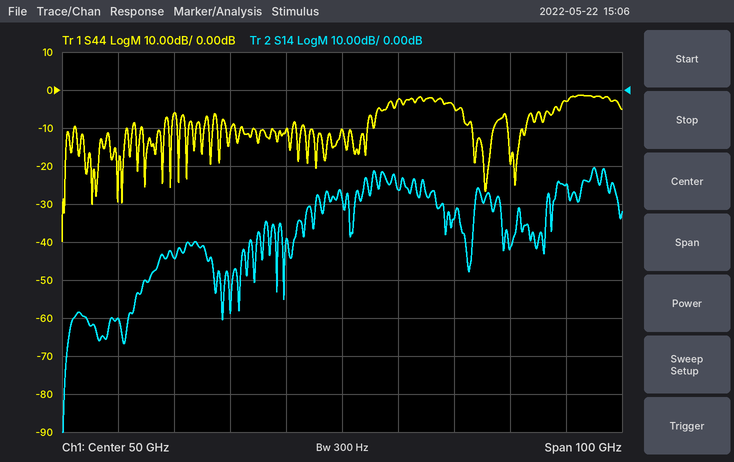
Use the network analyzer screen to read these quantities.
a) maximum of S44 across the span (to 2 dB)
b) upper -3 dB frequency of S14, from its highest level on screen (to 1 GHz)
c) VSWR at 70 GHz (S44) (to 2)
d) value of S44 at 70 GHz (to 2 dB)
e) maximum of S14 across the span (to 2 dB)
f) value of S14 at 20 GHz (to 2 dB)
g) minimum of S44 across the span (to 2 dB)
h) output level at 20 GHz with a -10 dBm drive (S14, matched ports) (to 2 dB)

-2 dB
96 GHz
4
-4 dB
-20 dB
-44 dB
-40 dB
-54 dBm
